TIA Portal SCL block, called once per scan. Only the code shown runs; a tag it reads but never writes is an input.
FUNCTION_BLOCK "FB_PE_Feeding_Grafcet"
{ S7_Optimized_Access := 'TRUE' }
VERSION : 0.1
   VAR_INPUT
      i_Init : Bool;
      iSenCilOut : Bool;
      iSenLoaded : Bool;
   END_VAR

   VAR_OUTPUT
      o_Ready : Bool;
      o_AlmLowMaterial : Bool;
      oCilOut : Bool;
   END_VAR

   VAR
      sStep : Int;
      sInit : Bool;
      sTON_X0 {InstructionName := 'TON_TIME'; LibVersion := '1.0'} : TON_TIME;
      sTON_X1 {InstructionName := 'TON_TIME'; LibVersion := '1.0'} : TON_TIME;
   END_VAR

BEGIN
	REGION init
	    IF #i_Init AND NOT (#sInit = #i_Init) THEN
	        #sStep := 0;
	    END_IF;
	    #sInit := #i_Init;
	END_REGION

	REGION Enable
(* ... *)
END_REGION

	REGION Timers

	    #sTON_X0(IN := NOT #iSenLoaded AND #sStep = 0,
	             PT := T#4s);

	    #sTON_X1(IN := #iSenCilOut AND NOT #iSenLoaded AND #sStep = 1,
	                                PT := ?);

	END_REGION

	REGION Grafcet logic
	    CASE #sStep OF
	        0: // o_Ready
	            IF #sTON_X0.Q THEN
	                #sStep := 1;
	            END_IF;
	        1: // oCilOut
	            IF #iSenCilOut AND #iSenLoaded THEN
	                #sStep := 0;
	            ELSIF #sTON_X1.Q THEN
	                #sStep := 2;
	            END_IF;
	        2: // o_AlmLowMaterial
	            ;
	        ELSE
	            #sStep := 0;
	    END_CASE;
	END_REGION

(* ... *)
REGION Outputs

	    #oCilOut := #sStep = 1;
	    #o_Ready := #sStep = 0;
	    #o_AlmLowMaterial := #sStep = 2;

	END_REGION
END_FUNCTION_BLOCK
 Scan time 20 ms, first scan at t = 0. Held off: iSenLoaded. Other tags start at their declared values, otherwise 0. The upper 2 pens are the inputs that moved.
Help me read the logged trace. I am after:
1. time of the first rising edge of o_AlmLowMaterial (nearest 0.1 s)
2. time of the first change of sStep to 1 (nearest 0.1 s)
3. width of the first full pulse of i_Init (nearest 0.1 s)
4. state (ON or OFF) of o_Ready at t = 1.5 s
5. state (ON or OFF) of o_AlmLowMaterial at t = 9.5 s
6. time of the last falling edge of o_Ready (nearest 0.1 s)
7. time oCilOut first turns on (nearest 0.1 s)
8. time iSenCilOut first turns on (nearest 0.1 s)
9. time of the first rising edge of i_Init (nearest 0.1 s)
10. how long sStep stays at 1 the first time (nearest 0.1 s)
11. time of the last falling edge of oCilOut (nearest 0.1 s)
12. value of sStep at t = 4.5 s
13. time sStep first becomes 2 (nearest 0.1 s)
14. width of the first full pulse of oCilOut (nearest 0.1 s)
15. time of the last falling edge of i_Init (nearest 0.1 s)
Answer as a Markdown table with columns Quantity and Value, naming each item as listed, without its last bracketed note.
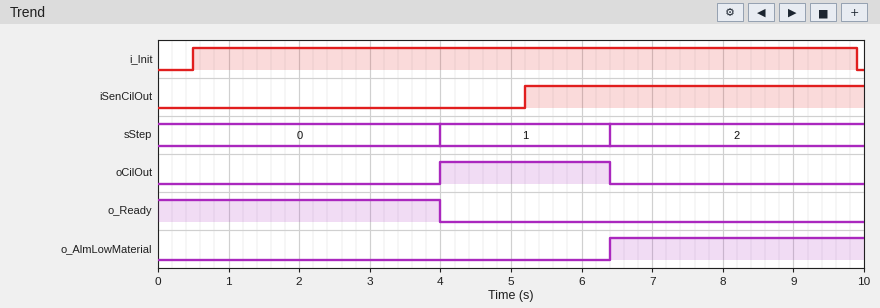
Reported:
| Quantity | Value |
|---|---|
| time of the first rising edge of o_AlmLowMaterial | 6.4 s |
| time of the first change of sStep to 1 | 4.0 s |
| width of the first full pulse of i_Init | 9.4 s |
| state (ON or OFF) of o_Ready at t = 1.5 s | ON |
| state (ON or OFF) of o_AlmLowMaterial at t = 9.5 s | ON |
| time of the last falling edge of o_Ready | 4.0 s |
| time oCilOut first turns on | 4.0 s |
| time iSenCilOut first turns on | 5.2 s |
| time of the first rising edge of i_Init | 0.5 s |
| how long sStep stays at 1 the first time | 2.4 s |
| time of the last falling edge of oCilOut | 6.4 s |
| value of sStep at t = 4.5 s | 1 |
| time sStep first becomes 2 | 6.4 s |
| width of the first full pulse of oCilOut | 2.4 s |
| time of the last falling edge of i_Init | 9.9 s |
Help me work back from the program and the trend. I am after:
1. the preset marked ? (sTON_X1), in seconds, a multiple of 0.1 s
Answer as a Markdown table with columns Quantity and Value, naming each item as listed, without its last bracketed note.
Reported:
| Quantity | Value |
|---|---|
| the preset marked ? (sTON_X1), in seconds, a multiple of 0.1 s | 1.2 s |
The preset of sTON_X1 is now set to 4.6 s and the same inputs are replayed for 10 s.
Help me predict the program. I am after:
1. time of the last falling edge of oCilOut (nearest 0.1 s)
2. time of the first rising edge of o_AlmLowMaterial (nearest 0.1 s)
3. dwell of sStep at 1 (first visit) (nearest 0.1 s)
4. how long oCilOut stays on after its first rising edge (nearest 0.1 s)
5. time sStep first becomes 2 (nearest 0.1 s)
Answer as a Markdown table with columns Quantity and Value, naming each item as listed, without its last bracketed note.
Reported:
| Quantity | Value |
|---|---|
| time of the last falling edge of oCilOut | 9.8 s |
| time of the first rising edge of o_AlmLowMaterial | 9.8 s |
| dwell of sStep at 1 (first visit) | 5.8 s |
| how long oCilOut stays on after its first rising edge | 5.8 s |
| time sStep first becomes 2 | 9.8 s |
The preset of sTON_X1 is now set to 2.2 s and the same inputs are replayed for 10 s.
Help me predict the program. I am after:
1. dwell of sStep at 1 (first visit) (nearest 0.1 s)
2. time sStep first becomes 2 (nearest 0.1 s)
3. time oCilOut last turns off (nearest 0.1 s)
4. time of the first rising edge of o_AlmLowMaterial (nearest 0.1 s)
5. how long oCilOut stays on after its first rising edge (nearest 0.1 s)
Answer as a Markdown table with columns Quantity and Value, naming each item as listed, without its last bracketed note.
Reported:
| Quantity | Value |
|---|---|
| dwell of sStep at 1 (first visit) | 3.4 s |
| time sStep first becomes 2 | 7.4 s |
| time oCilOut last turns off | 7.4 s |
| time of the first rising edge of o_AlmLowMaterial | 7.4 s |
| how long oCilOut stays on after its first rising edge | 3.4 s |
